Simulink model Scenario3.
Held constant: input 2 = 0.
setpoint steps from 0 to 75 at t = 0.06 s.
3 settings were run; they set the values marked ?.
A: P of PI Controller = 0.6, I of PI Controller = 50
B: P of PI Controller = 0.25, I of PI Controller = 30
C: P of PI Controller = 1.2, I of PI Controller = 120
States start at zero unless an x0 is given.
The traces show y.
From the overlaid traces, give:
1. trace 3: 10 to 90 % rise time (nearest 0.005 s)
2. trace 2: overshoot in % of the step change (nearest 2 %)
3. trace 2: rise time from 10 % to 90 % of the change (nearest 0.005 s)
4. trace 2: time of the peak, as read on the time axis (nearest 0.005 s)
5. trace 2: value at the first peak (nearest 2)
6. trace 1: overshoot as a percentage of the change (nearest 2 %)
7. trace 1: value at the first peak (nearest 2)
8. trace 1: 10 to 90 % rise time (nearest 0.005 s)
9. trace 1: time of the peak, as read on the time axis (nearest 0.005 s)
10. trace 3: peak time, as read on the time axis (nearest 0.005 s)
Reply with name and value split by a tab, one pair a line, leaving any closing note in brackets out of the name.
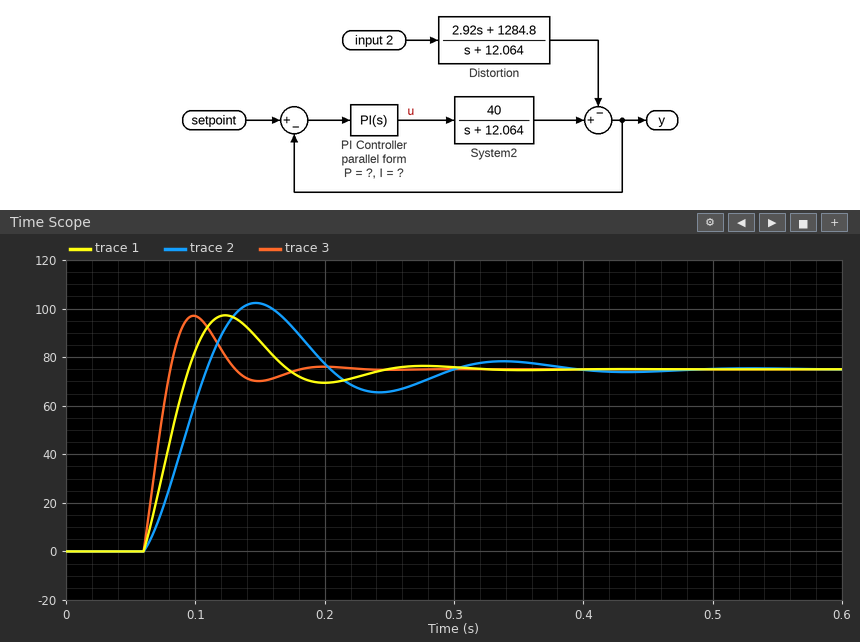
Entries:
trace 3: 10 to 90 % rise time	0.015 s
trace 2: overshoot in % of the step change	36 %
trace 2: rise time from 10 % to 90 % of the change	0.035 s
trace 2: time of the peak, as read on the time axis	0.145 s
trace 2: value at the first peak	102
trace 1: overshoot as a percentage of the change	30 %
trace 1: value at the first peak	98
trace 1: 10 to 90 % rise time	0.025 s
trace 1: time of the peak, as read on the time axis	0.125 s
trace 3: peak time, as read on the time axis	0.100 s
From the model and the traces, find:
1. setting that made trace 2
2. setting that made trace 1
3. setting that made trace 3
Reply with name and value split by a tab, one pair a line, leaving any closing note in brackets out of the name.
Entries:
setting that made trace 2	B
setting that made trace 1	A
setting that made trace 3	C
